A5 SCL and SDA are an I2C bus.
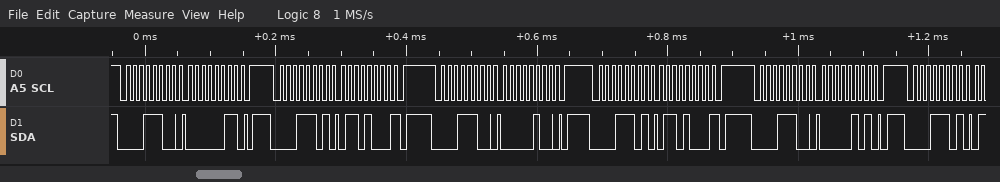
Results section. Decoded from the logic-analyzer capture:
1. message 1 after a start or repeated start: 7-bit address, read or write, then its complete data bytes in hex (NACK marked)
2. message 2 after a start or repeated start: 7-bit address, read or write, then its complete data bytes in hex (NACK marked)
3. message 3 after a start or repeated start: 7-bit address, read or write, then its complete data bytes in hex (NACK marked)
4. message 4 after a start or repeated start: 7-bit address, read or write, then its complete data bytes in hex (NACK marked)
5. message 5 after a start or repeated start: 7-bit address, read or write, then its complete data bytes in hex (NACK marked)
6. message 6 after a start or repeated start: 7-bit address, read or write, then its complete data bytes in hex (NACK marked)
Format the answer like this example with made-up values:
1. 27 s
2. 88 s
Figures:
1. 0x0E write: 03
2. 0x0E read: 68 NACK
3. 0x0E write: 04
4. 0x0E read: 68 NACK
5. 0x0E write: 05
6. 0x0E read
